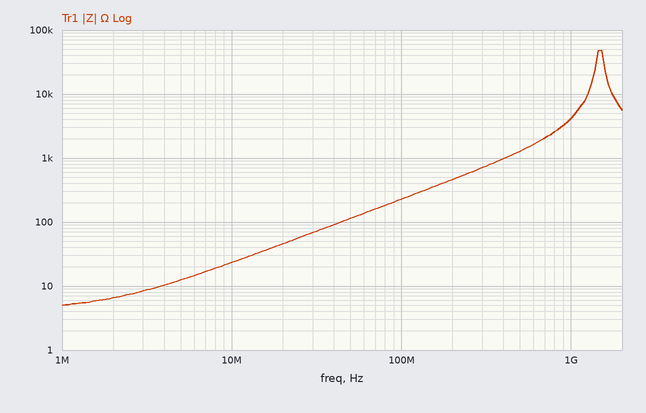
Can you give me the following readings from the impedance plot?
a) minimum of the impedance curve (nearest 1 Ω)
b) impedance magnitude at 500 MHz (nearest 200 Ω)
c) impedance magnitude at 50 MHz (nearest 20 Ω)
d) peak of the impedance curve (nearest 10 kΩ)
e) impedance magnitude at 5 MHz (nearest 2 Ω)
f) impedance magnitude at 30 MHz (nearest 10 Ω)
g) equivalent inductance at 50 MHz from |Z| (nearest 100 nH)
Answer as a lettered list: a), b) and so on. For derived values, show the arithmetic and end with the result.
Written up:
a) 5 Ω
b) 1.2 kΩ
c) 120 Ω
d) 50 kΩ
e) 12 Ω
f) 70 Ω
g) L = 120 Ω/(2π × 50 MHz) ≈ 382 nH, so 400 nH to the nearest 100 nH
